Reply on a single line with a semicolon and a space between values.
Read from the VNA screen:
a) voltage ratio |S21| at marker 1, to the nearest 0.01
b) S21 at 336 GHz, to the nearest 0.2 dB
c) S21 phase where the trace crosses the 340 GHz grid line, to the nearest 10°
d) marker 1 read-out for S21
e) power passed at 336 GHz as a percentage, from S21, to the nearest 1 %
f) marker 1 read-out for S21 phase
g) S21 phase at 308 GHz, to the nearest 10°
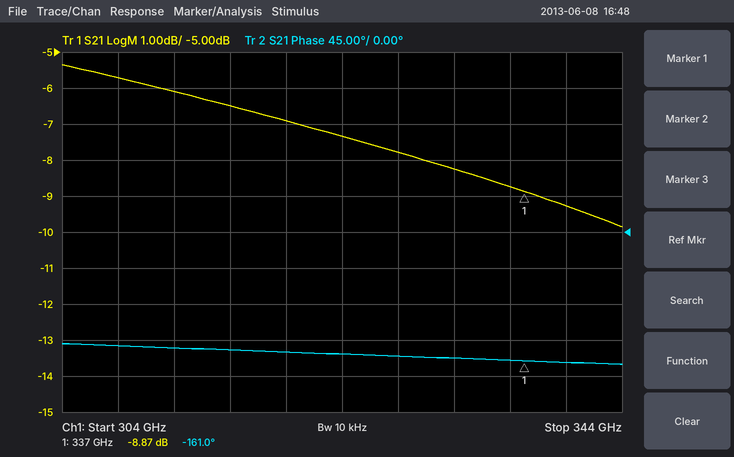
0.36; -8.8 dB; -160°; -8.87 dB; 13 %; -161.0°; -140°
